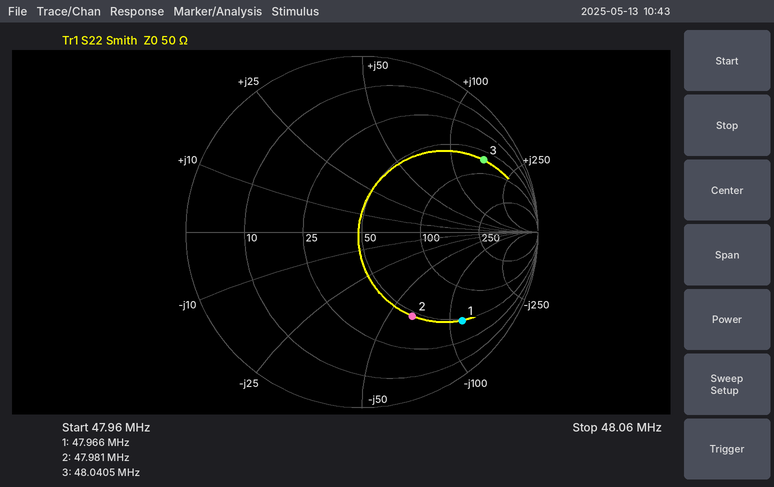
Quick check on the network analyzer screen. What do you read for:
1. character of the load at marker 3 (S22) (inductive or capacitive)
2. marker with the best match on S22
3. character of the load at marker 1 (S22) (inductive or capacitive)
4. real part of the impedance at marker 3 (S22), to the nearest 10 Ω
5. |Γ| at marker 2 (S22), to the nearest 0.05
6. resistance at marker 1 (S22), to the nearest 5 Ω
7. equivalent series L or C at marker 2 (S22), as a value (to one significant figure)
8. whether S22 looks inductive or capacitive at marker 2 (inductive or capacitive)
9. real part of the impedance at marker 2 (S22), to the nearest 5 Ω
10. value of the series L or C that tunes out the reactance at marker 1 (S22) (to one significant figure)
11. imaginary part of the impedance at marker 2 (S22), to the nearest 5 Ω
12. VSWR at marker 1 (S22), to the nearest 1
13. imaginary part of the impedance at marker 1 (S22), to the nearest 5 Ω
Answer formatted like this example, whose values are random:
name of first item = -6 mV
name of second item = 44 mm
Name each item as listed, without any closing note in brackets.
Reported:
character of the load at marker 3 (S22) = inductive
marker with the best match on S22 = marker 2
character of the load at marker 1 (S22) = capacitive
real part of the impedance at marker 3 (S22), to the nearest 10 Ω = 70 Ω
|Γ| at marker 2 (S22), to the nearest 0.05 = 0.55
resistance at marker 1 (S22), to the nearest 5 Ω = 50 Ω
equivalent series L or C at marker 2 (S22), as a value = 50 pF
whether S22 looks inductive or capacitive at marker 2 = capacitive
real part of the impedance at marker 2 (S22), to the nearest 5 Ω = 45 Ω
value of the series L or C that tunes out the reactance at marker 1 (S22) = 400 nH
imaginary part of the impedance at marker 2 (S22), to the nearest 5 Ω = -65 Ω
VSWR at marker 1 (S22), to the nearest 1 = 7
imaginary part of the impedance at marker 1 (S22), to the nearest 5 Ω = -115 Ω
